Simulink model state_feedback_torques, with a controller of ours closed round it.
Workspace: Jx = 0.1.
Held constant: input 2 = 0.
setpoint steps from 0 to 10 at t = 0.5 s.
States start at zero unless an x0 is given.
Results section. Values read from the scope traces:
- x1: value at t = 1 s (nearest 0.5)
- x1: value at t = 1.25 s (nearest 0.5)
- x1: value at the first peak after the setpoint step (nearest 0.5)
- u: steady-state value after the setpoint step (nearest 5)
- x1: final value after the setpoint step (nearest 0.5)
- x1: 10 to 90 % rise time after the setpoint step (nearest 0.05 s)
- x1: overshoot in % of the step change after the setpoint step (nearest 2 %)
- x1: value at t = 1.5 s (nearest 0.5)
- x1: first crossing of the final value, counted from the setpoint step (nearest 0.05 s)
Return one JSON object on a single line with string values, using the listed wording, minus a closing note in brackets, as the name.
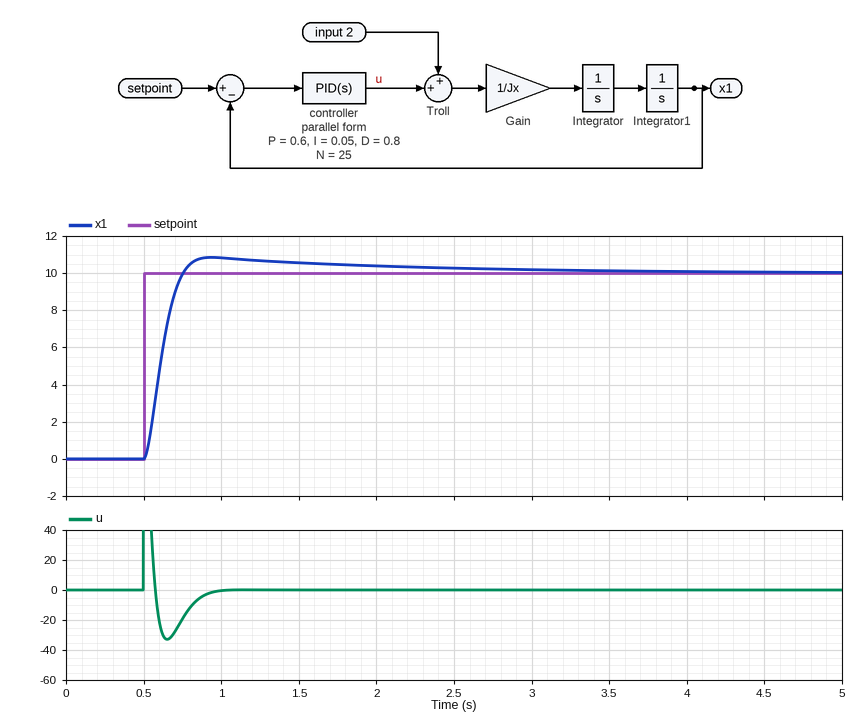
{"x1: value at t = 1 s": "11.0", "x1: value at t = 1.25 s": "10.5", "x1: value at the first peak after the setpoint step": "11.0", "u: steady-state value after the setpoint step": "0", "x1: final value after the setpoint step": "10.0", "x1: 10 to 90 % rise time after the setpoint step": "0.15 s", "x1: overshoot in % of the step change after the setpoint step": "8 %", "x1: value at t = 1.5 s": "10.5", "x1: first crossing of the final value, counted from the setpoint step": "0.25 s"}
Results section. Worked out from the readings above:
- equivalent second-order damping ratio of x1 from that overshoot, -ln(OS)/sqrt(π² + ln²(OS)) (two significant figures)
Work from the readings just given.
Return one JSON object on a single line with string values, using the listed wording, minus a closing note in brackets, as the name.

{"equivalent second-order damping ratio of x1 from that overshoot, -ln(OS)/sqrt(π² + ln²(OS))": "0.63"}
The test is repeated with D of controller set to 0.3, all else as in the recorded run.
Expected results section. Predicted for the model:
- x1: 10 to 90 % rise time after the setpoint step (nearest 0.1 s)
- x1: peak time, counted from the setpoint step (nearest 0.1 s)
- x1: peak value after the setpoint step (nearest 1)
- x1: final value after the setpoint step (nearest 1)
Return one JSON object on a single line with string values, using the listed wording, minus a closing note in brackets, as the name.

{"x1: 10 to 90 % rise time after the setpoint step": "0.3 s", "x1: peak time, counted from the setpoint step": "0.9 s", "x1: peak value after the setpoint step": "13", "x1: final value after the setpoint step": "10"}
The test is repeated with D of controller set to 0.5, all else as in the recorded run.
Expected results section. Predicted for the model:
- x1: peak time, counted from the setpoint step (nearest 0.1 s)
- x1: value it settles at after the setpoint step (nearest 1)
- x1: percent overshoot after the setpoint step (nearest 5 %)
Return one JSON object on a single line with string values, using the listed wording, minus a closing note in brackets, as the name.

{"x1: peak time, counted from the setpoint step": "0.7 s", "x1: value it settles at after the setpoint step": "10", "x1: percent overshoot after the setpoint step": "15 %"}
